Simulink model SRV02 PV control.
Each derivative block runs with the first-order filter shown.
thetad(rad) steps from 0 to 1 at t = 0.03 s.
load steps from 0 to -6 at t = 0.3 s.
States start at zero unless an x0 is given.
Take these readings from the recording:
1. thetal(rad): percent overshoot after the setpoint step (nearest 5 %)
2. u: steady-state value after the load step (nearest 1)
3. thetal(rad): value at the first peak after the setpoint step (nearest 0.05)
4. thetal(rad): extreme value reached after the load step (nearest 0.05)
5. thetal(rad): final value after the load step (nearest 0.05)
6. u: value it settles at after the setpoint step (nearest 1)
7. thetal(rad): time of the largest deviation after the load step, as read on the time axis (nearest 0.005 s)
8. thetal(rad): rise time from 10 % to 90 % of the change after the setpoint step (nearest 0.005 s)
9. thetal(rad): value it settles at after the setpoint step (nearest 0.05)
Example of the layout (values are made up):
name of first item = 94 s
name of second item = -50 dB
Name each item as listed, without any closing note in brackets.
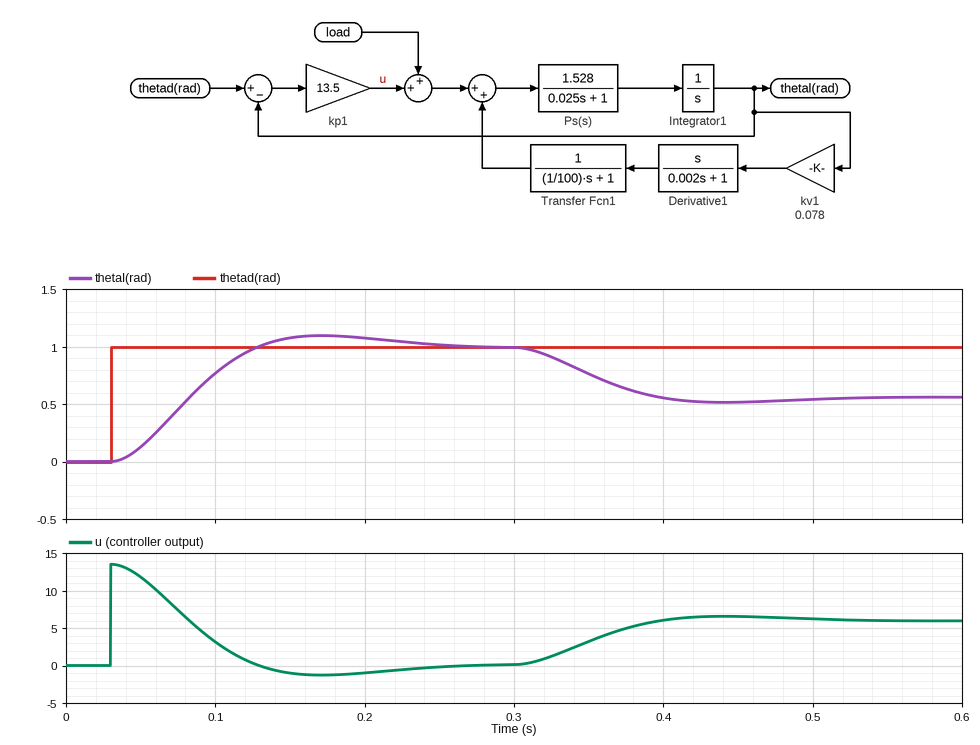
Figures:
thetal(rad): percent overshoot after the setpoint step = 10 %
u: steady-state value after the load step = 6
thetal(rad): value at the first peak after the setpoint step = 1.10
thetal(rad): extreme value reached after the load step = 0.50
thetal(rad): final value after the load step = 0.55
u: value it settles at after the setpoint step = 0
thetal(rad): time of the largest deviation after the load step, as read on the time axis = 0.440 s
thetal(rad): rise time from 10 % to 90 % of the change after the setpoint step = 0.065 s
thetal(rad): value it settles at after the setpoint step = 1.00
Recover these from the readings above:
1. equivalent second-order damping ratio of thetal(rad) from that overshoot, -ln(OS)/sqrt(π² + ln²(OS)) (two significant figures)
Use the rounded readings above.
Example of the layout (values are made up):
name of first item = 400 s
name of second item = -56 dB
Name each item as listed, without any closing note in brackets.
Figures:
equivalent second-order damping ratio of thetal(rad) from that overshoot, -ln(OS)/sqrt(π² + ln²(OS)) = 0.59
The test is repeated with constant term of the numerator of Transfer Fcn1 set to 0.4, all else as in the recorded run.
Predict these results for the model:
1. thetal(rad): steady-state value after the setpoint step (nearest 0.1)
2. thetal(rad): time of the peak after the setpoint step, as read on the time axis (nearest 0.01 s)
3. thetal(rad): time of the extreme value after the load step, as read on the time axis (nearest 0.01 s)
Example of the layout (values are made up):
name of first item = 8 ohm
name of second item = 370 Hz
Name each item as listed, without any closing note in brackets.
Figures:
thetal(rad): steady-state value after the setpoint step = 1.0
thetal(rad): time of the peak after the setpoint step, as read on the time axis = 0.18 s
thetal(rad): time of the extreme value after the load step, as read on the time axis = 0.45 s
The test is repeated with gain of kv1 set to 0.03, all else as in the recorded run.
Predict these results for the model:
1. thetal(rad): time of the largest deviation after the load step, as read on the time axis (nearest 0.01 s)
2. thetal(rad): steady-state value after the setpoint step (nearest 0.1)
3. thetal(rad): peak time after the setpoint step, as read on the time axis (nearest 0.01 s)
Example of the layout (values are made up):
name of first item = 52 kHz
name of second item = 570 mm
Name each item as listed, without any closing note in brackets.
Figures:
thetal(rad): time of the largest deviation after the load step, as read on the time axis = 0.45 s
thetal(rad): steady-state value after the setpoint step = 1.0
thetal(rad): peak time after the setpoint step, as read on the time axis = 0.18 s
